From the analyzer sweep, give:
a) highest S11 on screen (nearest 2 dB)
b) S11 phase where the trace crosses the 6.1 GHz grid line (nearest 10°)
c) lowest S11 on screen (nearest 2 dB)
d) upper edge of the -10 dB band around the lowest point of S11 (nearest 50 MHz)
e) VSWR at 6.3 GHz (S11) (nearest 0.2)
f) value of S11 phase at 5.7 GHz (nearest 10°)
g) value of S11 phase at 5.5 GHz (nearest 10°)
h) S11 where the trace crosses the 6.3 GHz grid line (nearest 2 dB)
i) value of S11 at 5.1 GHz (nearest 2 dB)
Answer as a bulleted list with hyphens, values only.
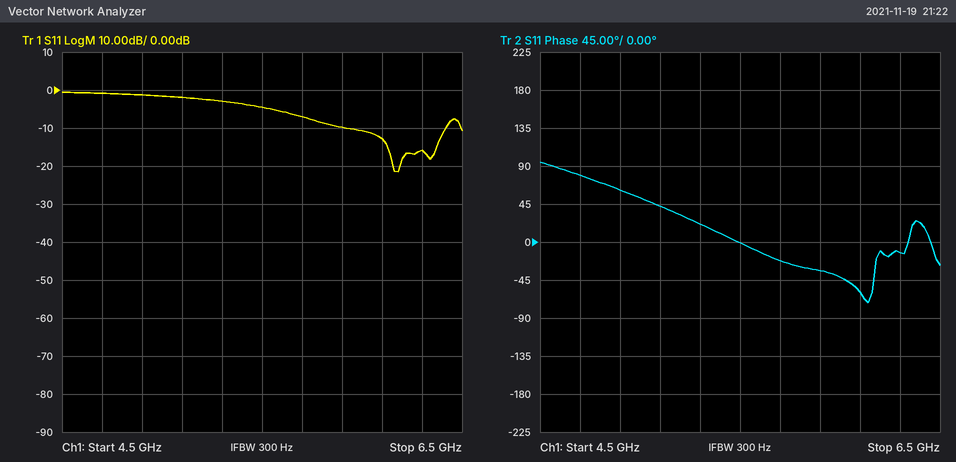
- 0 dB
- -60°
- -22 dB
- 6.40 GHz
- 1.4
- -20°
- 0°
- -16 dB
- -2 dB
